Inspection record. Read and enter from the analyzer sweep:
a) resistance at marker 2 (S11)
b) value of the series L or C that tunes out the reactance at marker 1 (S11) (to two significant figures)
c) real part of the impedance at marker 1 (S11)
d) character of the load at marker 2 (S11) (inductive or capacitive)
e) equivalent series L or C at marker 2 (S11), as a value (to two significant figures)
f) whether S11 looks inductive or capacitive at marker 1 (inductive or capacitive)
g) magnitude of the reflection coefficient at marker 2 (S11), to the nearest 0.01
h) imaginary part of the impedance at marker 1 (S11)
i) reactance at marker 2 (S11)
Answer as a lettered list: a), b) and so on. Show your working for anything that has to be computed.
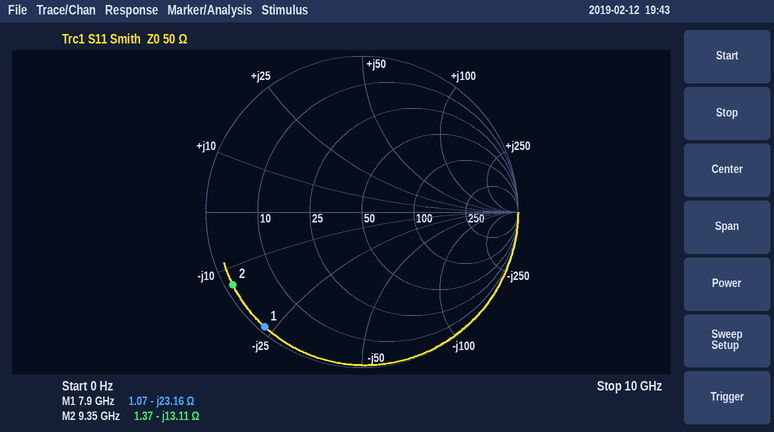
a) 1.37 Ω
b) L = 23.16 Ω/(2π × 7.9 GHz) ≈ 467 pH, so 470 pH to two significant figures
c) 1.07 Ω
d) capacitive
e) C = 1/(2π × 9.35 GHz × 13.11 Ω) ≈ 1.3 pF
f) capacitive
g) 0.95
h) -23.16 Ω
i) -13.11 Ω
